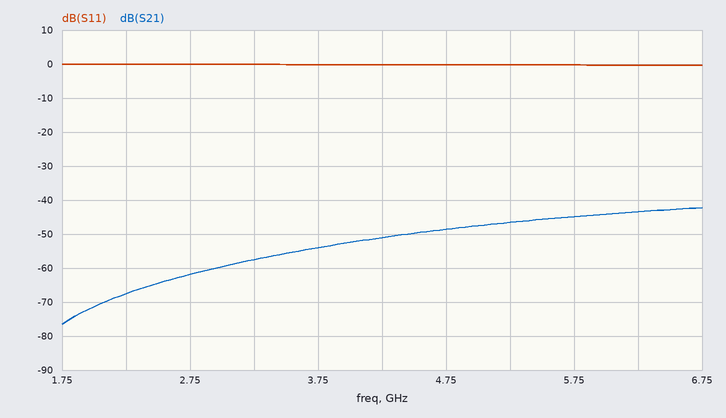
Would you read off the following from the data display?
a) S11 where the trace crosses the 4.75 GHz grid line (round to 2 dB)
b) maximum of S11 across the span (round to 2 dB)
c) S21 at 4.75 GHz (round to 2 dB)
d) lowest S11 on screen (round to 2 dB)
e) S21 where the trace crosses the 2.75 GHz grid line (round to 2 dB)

0 dB
0 dB
-48 dB
0 dB
-62 dB
